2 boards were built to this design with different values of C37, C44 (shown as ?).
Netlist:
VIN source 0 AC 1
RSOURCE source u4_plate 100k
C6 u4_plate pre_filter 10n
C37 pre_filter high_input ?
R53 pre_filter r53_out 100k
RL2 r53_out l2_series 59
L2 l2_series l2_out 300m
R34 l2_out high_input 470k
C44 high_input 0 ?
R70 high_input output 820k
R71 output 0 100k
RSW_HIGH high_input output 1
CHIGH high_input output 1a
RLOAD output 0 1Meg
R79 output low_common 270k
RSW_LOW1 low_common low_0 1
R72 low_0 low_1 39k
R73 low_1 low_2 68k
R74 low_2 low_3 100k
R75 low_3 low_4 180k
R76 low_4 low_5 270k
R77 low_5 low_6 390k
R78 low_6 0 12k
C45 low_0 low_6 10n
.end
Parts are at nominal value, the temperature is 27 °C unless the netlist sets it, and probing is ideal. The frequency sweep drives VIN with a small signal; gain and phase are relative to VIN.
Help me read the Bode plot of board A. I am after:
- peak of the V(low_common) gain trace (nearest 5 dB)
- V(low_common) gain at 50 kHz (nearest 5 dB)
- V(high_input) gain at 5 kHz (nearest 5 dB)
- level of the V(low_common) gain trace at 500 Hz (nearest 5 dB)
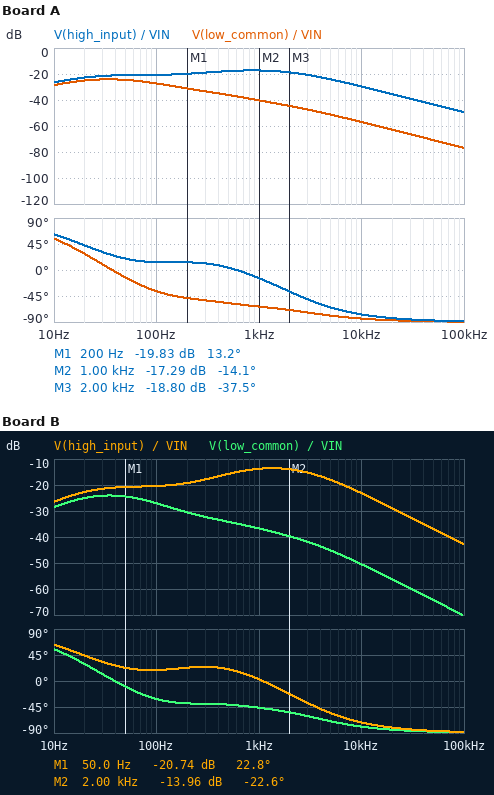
-25 dB
-70 dB
-25 dB
-35 dB
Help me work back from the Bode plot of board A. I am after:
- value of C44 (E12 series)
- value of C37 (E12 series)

4.7 nF
1.2 nF
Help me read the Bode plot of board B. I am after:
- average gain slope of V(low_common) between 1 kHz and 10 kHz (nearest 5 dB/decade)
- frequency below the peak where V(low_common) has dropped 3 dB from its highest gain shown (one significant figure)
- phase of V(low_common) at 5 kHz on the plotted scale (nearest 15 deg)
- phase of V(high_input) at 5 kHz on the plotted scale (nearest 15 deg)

-15 dB/decade
10 Hz
-75 deg
-60 deg
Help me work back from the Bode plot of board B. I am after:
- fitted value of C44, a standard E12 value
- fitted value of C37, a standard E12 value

2.2 nF
1.2 nF
